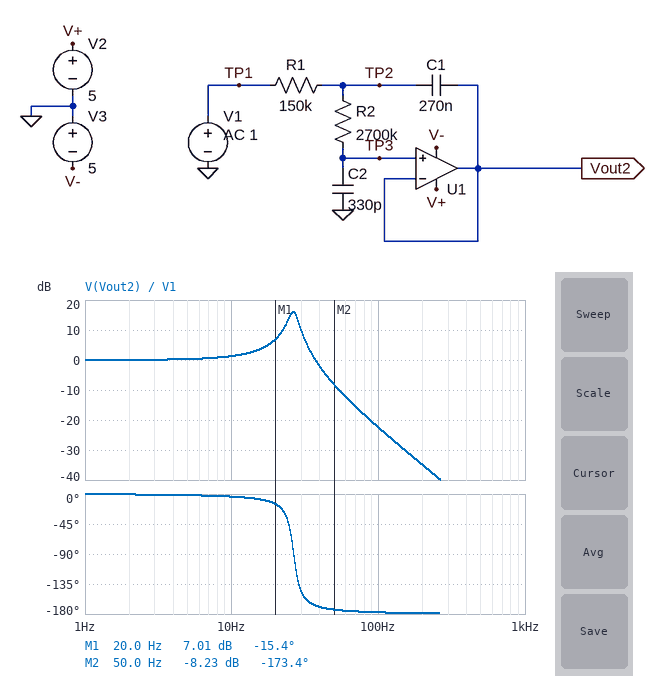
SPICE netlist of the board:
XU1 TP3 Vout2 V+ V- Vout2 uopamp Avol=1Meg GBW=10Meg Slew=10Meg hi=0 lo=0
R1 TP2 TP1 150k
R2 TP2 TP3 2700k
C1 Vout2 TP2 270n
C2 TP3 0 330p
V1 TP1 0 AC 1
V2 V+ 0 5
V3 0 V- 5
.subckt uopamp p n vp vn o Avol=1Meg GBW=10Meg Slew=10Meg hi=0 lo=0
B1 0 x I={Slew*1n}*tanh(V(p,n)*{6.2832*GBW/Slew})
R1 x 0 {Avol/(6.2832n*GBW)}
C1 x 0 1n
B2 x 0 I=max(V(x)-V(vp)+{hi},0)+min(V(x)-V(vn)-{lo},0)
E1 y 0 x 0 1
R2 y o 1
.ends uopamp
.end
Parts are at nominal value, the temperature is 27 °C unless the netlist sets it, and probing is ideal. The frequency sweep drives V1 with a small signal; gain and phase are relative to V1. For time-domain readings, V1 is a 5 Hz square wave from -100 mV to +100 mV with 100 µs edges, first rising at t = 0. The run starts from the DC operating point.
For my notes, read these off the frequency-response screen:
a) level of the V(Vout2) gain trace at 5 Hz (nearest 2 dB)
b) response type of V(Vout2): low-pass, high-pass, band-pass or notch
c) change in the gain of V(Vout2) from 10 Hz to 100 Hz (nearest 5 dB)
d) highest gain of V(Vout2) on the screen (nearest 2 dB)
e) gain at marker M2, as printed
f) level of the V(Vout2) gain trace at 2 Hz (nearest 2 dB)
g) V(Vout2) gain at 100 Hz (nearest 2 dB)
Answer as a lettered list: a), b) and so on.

a) 0 dB
b) low-pass
c) -25 dB
d) 16 dB
e) -8.23 dB
f) 0 dB
g) -22 dB
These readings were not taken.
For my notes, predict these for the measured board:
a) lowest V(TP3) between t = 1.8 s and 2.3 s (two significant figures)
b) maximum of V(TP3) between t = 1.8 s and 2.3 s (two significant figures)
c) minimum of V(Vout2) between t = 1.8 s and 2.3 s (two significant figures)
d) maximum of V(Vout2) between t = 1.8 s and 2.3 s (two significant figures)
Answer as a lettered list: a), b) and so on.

a) -290 mV
b) 290 mV
c) -290 mV
d) 290 mV
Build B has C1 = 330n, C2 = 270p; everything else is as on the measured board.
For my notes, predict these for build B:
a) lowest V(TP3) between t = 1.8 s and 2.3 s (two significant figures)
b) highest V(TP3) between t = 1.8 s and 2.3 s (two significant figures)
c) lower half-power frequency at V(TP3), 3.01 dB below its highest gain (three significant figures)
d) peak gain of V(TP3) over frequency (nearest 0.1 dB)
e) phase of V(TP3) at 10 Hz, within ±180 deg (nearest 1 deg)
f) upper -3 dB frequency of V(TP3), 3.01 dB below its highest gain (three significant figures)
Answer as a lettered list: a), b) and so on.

a) -300 mV
b) 300 mV
c) 24.6 Hz
d) 17.9 dB
e) -3 deg
f) 28.0 Hz
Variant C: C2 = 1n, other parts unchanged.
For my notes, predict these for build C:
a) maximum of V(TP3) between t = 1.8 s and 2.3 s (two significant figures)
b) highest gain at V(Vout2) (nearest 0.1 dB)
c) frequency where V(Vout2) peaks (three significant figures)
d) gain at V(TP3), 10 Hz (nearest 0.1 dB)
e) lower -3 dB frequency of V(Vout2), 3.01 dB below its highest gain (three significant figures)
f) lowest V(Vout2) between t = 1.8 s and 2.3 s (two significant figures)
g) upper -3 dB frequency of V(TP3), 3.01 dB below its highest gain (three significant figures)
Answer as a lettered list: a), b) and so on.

a) 280 mV
b) 11.4 dB
c) 14.9 Hz
d) 4.5 dB
e) 12.7 Hz
f) -280 mV
g) 16.9 Hz
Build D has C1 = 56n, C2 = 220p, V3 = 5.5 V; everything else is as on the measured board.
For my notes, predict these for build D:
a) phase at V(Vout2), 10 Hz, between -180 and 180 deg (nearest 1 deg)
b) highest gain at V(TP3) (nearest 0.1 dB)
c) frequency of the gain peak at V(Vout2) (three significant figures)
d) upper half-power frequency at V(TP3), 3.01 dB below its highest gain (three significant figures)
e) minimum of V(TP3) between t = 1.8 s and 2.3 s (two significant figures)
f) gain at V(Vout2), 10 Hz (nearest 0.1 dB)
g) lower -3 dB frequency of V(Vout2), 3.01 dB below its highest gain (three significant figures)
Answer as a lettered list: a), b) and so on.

a) -2 deg
b) 11.1 dB
c) 69.8 Hz
d) 79.3 Hz
e) -230 mV
f) 0.2 dB
g) 58.9 Hz
